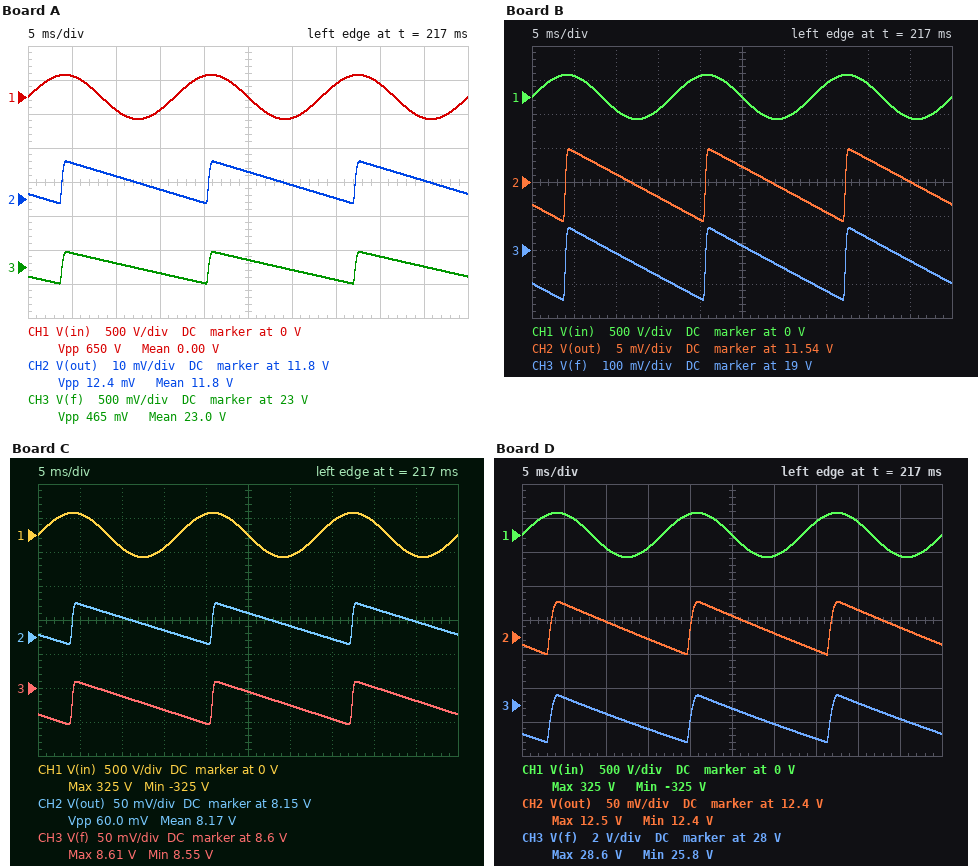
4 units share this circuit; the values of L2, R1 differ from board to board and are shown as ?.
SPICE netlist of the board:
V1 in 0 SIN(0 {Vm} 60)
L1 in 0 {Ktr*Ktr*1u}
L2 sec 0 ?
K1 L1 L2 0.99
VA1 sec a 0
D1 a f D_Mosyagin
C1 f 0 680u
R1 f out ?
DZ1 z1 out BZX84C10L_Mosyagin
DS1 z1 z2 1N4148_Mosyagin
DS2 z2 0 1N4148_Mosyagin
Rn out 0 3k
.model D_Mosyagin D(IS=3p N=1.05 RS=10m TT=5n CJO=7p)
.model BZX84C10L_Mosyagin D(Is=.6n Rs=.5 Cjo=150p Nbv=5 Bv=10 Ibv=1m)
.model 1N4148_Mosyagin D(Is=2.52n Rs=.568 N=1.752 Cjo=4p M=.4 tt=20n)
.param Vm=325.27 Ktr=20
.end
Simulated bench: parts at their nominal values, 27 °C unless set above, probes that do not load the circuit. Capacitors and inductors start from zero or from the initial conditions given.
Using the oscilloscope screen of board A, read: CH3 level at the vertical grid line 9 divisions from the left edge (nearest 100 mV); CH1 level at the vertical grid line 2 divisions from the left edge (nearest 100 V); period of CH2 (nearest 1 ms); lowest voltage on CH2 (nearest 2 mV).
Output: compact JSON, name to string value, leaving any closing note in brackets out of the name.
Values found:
{"CH3 level at the vertical grid line 9 divisions from the left edge": "23.0 V", "CH1 level at the vertical grid line 2 divisions from the left edge": "-200 V", "period of CH2": "17 ms", "lowest voltage on CH2": "11.798 V"}
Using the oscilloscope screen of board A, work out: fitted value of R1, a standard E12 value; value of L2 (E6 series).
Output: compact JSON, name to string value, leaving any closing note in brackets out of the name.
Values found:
{"fitted value of R1, a standard E12 value": "560 Ω", "value of L2": "2.2 µH"}
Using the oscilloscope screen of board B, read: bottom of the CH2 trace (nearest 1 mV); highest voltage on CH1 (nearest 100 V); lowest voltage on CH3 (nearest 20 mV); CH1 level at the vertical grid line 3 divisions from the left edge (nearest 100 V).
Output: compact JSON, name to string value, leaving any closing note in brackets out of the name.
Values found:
{"bottom of the CH2 trace": "11.534 V", "highest voltage on CH1": "300 V", "lowest voltage on CH3": "18.86 V", "CH1 level at the vertical grid line 3 divisions from the left edge": "-200 V"}
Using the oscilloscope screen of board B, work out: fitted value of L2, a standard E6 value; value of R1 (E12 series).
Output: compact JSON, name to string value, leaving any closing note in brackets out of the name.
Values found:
{"fitted value of L2, a standard E6 value": "1.5 µH", "value of R1": "820 Ω"}
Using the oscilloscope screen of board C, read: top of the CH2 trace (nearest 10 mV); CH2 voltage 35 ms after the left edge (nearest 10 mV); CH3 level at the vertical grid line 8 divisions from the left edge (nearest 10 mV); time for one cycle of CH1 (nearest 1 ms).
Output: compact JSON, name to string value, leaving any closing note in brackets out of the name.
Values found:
{"top of the CH2 trace": "8.20 V", "CH2 voltage 35 ms after the left edge": "8.15 V", "CH3 level at the vertical grid line 8 divisions from the left edge": "8.60 V", "time for one cycle of CH1": "17 ms"}
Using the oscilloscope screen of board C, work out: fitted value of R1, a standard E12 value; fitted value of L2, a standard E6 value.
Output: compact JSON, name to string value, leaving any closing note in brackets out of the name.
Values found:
{"fitted value of R1, a standard E12 value": "150 Ω", "fitted value of L2, a standard E6 value": "330 nH"}
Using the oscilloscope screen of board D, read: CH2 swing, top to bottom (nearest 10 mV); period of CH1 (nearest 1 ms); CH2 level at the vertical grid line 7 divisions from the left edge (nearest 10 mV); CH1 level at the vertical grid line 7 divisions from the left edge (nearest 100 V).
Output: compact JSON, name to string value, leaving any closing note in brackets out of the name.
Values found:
{"CH2 swing, top to bottom": "80 mV", "period of CH1": "17 ms", "CH2 level at the vertical grid line 7 divisions from the left edge": "12.38 V", "CH1 level at the vertical grid line 7 divisions from the left edge": "200 V"}
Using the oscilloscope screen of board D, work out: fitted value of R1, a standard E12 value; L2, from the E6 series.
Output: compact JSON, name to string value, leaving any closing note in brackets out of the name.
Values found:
{"fitted value of R1, a standard E12 value": "120 Ω", "L2, from the E6 series": "3.3 µH"}
